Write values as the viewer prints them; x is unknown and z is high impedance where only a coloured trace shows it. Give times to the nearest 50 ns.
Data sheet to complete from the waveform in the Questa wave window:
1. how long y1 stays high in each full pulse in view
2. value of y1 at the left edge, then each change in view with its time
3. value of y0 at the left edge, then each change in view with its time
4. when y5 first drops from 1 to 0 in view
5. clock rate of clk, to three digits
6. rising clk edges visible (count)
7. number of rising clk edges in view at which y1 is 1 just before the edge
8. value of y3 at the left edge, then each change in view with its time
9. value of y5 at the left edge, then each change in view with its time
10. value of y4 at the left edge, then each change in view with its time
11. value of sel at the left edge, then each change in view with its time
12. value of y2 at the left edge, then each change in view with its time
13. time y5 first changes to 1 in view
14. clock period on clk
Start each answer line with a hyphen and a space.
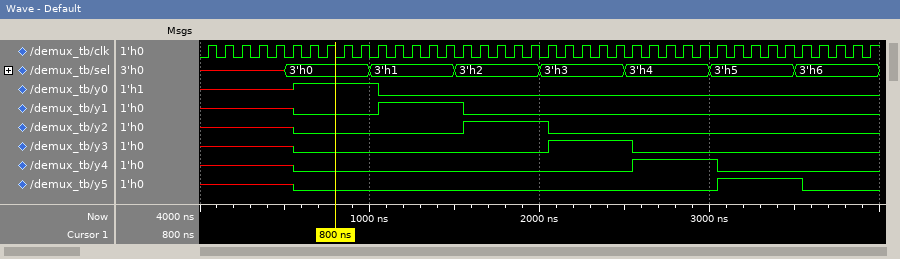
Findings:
- 500 ns
- x, 0 at 550 ns, 1 at 1050 ns, 0 at 1550 ns
- x, 1 at 550 ns, 0 at 1050 ns
- 3550 ns
- 10.0 MHz
- 40
- 5
- x, 0 at 550 ns, 1 at 2050 ns, 0 at 2550 ns
- x, 0 at 550 ns, 1 at 3050 ns, 0 at 3550 ns
- x, 0 at 550 ns, 1 at 2550 ns, 0 at 3050 ns
- x, 3'h0 at 500 ns, 3'h1 at 1000 ns, 3'h2 at 1500 ns, 3'h3 at 2000 ns, 3'h4 at 2500 ns, 3'h5 at 3000 ns, 3'h6 at 3500 ns
- x, 0 at 550 ns, 1 at 1550 ns, 0 at 2050 ns
- 3050 ns
- 100 ns
